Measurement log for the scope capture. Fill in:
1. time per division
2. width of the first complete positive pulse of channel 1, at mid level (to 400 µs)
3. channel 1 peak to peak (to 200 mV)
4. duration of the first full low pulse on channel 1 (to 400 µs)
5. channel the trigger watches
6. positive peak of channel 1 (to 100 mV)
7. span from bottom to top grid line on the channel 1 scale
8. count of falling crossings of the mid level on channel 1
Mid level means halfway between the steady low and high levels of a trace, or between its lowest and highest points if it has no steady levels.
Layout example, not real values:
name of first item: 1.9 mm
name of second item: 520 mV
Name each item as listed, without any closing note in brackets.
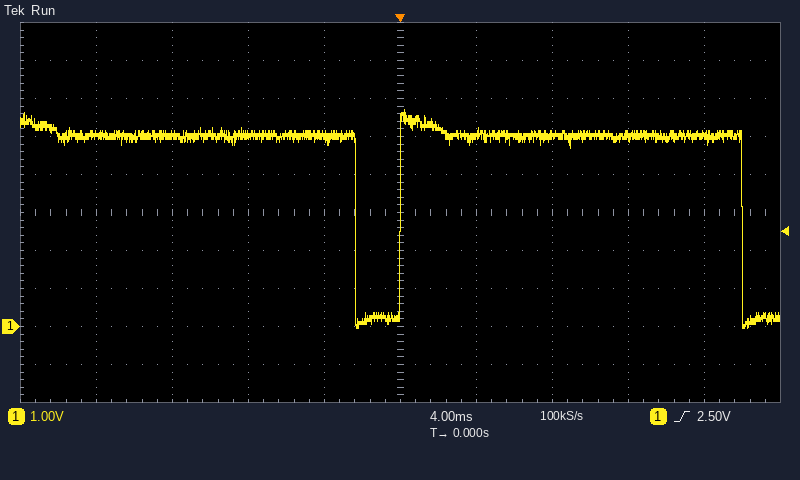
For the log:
time per division: 4 ms
width of the first complete positive pulse of channel 1, at mid level: 18.0 ms
channel 1 peak to peak: 5.8 V
duration of the first full low pulse on channel 1: 2.4 ms
channel the trigger watches: channel 1
positive peak of channel 1: 5.7 V
span from bottom to top grid line on the channel 1 scale: 10 V
count of falling crossings of the mid level on channel 1: 2
